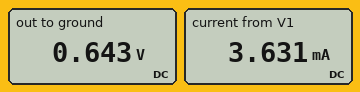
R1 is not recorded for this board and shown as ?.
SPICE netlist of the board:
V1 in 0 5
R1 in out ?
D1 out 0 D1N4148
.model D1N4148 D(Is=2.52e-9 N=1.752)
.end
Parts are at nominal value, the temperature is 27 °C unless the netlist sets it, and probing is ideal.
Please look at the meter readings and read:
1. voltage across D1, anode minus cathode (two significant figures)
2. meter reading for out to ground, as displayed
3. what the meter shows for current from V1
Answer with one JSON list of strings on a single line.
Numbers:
["640 mV", "0.643 V", "3.631 mA"]
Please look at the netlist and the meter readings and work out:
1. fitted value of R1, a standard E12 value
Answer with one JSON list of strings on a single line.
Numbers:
["1.2 kΩ"]
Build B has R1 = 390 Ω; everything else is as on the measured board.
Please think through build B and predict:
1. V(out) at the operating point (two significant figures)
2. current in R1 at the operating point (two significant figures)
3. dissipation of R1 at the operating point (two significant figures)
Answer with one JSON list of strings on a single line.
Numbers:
["690 mV", "11 mA", "48 mW"]
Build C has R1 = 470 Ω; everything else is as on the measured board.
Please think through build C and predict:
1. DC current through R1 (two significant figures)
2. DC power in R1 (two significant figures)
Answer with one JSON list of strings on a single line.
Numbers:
["9.2 mA", "40 mW"]
